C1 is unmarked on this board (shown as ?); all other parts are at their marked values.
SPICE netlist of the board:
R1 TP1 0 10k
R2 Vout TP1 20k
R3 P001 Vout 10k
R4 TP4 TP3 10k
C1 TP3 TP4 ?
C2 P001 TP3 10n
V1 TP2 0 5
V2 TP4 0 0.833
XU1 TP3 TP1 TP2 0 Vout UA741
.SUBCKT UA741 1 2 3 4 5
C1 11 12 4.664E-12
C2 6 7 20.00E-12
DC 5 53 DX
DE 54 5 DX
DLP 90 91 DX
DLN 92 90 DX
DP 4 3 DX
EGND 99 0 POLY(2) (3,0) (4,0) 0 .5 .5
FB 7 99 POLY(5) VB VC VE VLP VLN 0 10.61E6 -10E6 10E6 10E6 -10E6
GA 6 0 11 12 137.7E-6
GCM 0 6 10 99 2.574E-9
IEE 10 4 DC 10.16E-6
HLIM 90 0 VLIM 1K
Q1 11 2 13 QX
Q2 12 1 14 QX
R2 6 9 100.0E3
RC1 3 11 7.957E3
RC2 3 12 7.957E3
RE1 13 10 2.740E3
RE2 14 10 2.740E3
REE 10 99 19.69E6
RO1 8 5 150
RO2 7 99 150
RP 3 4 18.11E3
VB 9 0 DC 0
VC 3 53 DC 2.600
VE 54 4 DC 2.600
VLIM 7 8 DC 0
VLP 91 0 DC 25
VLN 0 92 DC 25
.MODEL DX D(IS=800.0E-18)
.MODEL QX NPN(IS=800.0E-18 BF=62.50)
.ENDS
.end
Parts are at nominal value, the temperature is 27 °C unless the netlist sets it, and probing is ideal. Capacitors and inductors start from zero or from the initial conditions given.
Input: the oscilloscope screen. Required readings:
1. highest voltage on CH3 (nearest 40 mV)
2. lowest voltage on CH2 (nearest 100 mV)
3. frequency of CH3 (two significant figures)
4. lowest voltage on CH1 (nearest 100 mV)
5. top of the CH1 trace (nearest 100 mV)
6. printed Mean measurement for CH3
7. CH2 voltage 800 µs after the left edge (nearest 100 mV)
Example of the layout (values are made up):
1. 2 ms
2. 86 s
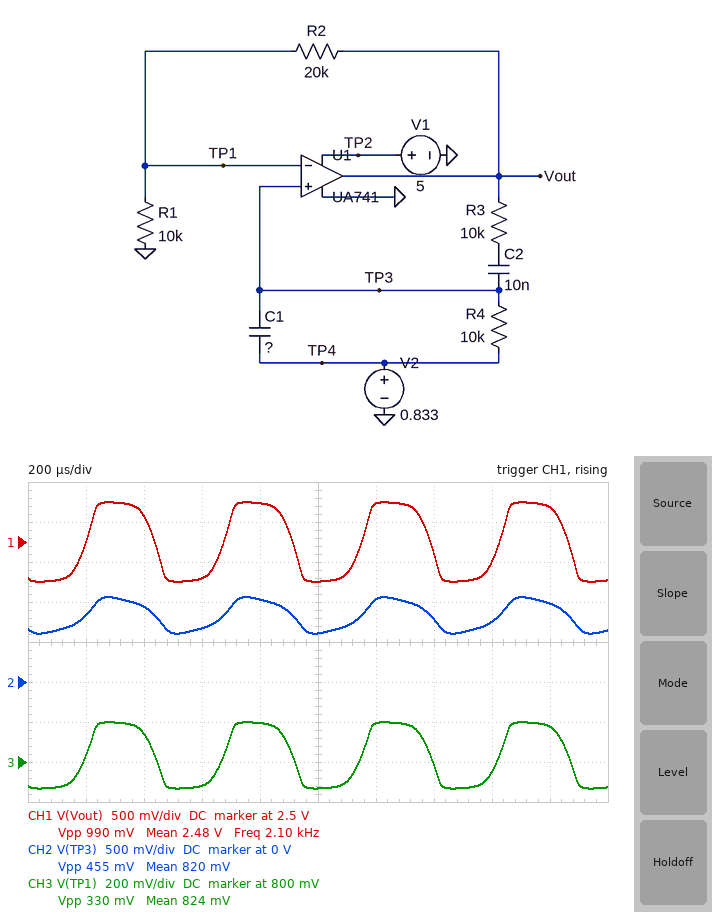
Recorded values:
1. 1.00 V
2. 600 mV
3. 2.1 kHz
4. 2.0 V
5. 3.0 V
6. 824 mV
7. 1.0 V
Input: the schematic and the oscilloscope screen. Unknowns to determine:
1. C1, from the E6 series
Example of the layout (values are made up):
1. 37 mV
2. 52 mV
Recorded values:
1. 4.7 nF
